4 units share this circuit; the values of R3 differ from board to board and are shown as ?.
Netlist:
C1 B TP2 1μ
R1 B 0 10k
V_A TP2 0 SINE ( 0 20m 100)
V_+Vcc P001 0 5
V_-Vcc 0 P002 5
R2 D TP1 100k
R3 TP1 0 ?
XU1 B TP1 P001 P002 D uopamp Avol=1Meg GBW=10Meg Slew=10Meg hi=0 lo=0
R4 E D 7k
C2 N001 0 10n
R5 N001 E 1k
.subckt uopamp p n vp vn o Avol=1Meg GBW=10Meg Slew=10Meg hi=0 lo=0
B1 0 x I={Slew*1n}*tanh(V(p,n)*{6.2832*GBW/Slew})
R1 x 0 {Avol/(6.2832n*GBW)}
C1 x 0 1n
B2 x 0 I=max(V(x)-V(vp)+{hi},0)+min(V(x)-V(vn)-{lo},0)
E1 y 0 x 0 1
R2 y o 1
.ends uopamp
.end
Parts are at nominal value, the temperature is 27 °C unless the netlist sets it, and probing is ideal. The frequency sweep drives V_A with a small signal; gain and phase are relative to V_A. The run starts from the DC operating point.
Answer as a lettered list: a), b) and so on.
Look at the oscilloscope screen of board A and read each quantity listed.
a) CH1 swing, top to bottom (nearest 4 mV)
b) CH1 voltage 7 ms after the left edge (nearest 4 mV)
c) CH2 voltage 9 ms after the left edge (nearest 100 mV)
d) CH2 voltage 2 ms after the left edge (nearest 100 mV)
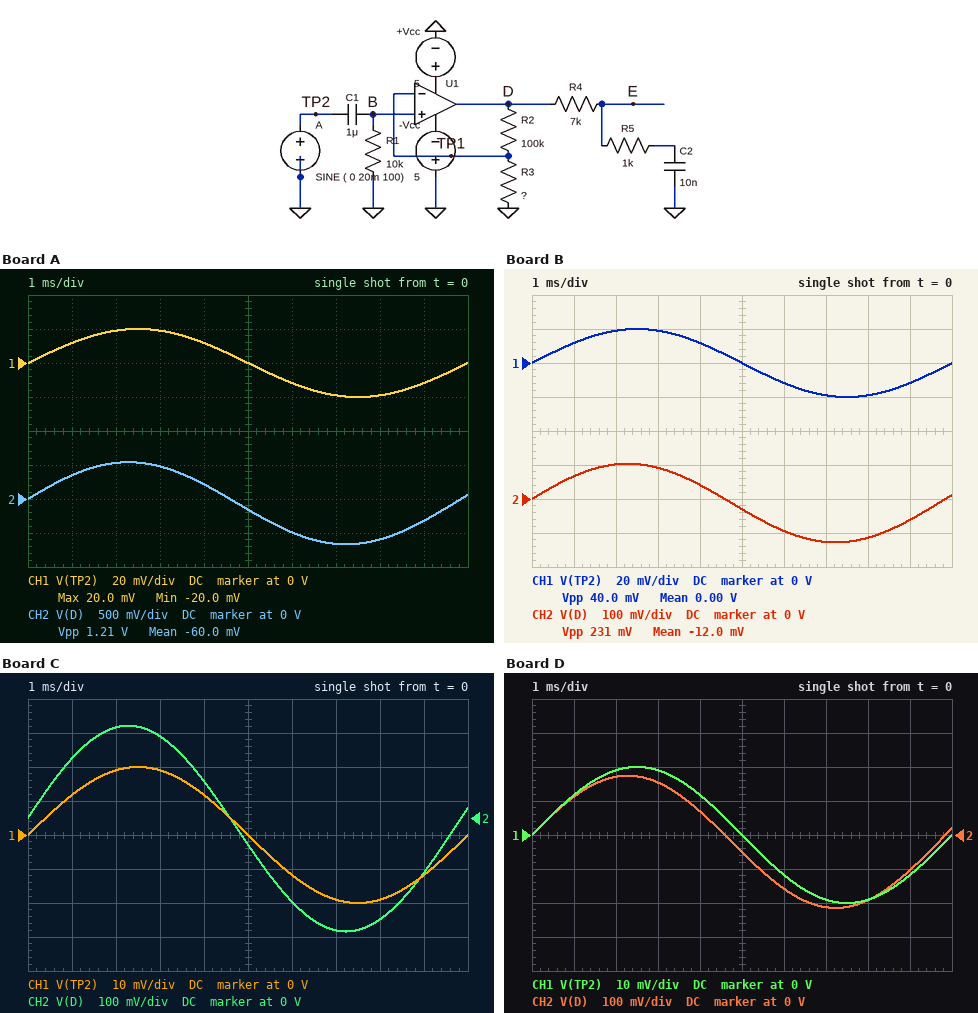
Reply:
a) 40 mV
b) -20 mV
c) -300 mV
d) 500 mV
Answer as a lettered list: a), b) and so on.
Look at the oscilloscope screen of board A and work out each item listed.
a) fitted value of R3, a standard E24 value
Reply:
a) 3.3 kΩ
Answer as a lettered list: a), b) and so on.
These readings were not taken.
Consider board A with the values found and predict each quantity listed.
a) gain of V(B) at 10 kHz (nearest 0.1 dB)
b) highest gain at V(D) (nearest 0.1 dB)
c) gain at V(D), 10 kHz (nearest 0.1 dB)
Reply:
a) 0 dB
b) 29.9 dB
c) 29.9 dB
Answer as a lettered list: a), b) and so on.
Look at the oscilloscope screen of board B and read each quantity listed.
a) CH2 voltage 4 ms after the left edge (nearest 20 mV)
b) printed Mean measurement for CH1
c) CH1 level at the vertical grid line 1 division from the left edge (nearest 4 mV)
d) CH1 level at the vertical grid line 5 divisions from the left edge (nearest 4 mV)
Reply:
a) 40 mV
b) 0.00 V
c) 12 mV
d) 0 V
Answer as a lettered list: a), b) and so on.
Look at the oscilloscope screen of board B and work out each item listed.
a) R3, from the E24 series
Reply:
a) 20 kΩ
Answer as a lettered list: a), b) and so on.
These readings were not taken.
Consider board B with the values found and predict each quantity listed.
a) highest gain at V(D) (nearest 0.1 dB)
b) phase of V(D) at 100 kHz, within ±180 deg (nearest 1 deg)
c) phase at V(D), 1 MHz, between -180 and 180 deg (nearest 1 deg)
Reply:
a) 15.6 dB
b) -3 deg
c) -31 deg
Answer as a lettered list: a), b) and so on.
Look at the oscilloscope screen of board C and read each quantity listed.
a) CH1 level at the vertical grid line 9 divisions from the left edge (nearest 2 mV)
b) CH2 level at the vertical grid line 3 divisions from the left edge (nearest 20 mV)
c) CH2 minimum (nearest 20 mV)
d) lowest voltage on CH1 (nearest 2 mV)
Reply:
a) -12 mV
b) 240 mV
c) -340 mV
d) -20 mV
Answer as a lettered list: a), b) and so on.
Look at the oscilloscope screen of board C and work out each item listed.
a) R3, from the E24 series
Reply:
a) 6.8 kΩ
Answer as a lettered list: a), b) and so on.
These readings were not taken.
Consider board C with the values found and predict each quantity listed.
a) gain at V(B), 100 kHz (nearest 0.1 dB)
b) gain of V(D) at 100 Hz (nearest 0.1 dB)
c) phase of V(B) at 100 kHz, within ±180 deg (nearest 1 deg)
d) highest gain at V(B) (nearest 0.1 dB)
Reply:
a) 0 dB
b) 23.8 dB
c) 0 deg
d) 0 dB
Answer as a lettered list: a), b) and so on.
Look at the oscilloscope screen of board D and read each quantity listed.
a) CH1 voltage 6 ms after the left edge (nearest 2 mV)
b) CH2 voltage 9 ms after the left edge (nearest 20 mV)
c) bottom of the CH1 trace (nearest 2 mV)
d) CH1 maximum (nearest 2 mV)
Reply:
a) -12 mV
b) -100 mV
c) -20 mV
d) 20 mV
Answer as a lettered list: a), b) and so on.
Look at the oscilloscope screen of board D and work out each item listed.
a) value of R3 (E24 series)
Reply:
a) 11 kΩ
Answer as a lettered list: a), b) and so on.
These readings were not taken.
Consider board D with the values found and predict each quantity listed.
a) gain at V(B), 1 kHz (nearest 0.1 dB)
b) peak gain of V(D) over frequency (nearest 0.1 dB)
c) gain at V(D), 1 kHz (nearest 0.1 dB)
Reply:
a) 0 dB
b) 20.1 dB
c) 20.1 dB
